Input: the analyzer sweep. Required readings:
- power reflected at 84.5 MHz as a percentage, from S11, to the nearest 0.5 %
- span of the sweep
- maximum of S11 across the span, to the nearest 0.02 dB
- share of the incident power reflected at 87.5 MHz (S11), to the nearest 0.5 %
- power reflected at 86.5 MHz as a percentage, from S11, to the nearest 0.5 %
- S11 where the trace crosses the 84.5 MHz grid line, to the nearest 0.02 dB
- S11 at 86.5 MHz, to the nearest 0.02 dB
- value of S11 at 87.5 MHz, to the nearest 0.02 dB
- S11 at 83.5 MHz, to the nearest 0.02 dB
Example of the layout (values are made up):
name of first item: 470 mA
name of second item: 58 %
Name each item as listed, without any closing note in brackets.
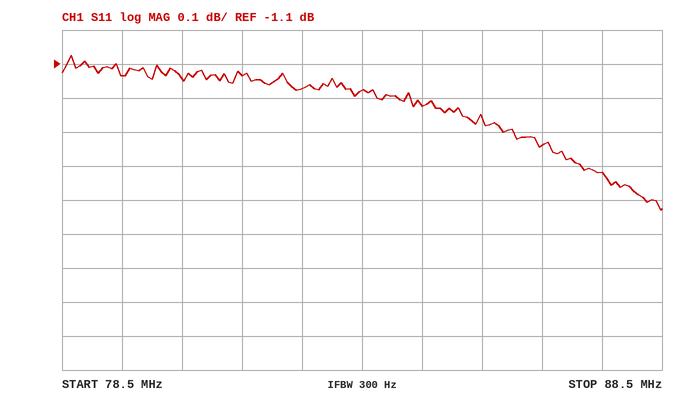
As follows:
power reflected at 84.5 MHz as a percentage, from S11, to the nearest 0.5 %: 75.5 %
span of the sweep: 10 MHz
maximum of S11 across the span, to the nearest 0.02 dB: -1.08 dB
share of the incident power reflected at 87.5 MHz (S11), to the nearest 0.5 %: 72.0 %
power reflected at 86.5 MHz as a percentage, from S11, to the nearest 0.5 %: 73.5 %
S11 where the trace crosses the 84.5 MHz grid line, to the nearest 0.02 dB: -1.22 dB
S11 at 86.5 MHz, to the nearest 0.02 dB: -1.34 dB
value of S11 at 87.5 MHz, to the nearest 0.02 dB: -1.42 dB
S11 at 83.5 MHz, to the nearest 0.02 dB: -1.18 dB
